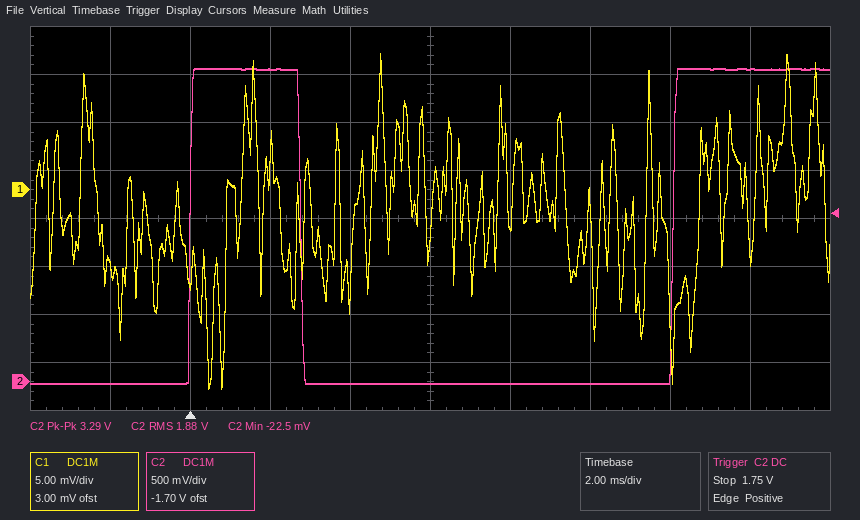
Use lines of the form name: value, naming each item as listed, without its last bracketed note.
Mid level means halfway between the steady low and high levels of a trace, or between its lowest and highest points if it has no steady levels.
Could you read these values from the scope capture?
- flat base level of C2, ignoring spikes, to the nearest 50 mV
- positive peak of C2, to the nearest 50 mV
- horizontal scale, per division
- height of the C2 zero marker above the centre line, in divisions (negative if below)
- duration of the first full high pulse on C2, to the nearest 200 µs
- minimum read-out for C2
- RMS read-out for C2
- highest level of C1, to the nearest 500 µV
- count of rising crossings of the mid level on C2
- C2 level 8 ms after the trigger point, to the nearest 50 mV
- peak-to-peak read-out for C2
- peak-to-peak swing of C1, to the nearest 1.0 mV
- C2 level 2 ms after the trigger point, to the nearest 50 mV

flat base level of C2, ignoring spikes, to the nearest 50 mV: 0 mV
positive peak of C2, to the nearest 50 mV: 3.25 V
horizontal scale, per division: 2 ms
height of the C2 zero marker above the centre line, in divisions: -3.4 div
duration of the first full high pulse on C2, to the nearest 200 µs: 2.8 ms
minimum read-out for C2: -22.5 mV
RMS read-out for C2: 1.88 V
highest level of C1, to the nearest 500 µV: 14.0 mV
count of rising crossings of the mid level on C2: 2
C2 level 8 ms after the trigger point, to the nearest 50 mV: 0 mV
peak-to-peak read-out for C2: 3.29 V
peak-to-peak swing of C1, to the nearest 1.0 mV: 35.0 mV
C2 level 2 ms after the trigger point, to the nearest 50 mV: 3.25 V
